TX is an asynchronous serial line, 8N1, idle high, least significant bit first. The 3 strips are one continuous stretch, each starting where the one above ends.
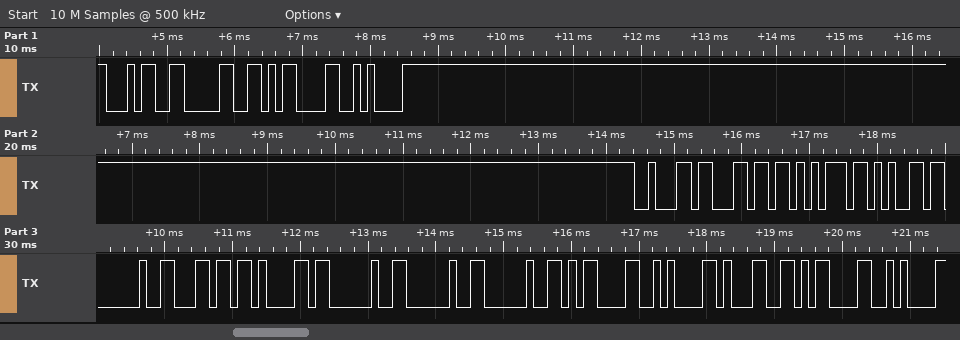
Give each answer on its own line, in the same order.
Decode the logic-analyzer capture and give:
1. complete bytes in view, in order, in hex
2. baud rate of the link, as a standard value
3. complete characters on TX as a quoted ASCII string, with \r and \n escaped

34 30 0D 0A 62 6C 75 65 20 6C 61 20 20 20 0D 0A 31 0D 0A
9600 baud
"40\r\nblue la   \r\n1\r\n"
